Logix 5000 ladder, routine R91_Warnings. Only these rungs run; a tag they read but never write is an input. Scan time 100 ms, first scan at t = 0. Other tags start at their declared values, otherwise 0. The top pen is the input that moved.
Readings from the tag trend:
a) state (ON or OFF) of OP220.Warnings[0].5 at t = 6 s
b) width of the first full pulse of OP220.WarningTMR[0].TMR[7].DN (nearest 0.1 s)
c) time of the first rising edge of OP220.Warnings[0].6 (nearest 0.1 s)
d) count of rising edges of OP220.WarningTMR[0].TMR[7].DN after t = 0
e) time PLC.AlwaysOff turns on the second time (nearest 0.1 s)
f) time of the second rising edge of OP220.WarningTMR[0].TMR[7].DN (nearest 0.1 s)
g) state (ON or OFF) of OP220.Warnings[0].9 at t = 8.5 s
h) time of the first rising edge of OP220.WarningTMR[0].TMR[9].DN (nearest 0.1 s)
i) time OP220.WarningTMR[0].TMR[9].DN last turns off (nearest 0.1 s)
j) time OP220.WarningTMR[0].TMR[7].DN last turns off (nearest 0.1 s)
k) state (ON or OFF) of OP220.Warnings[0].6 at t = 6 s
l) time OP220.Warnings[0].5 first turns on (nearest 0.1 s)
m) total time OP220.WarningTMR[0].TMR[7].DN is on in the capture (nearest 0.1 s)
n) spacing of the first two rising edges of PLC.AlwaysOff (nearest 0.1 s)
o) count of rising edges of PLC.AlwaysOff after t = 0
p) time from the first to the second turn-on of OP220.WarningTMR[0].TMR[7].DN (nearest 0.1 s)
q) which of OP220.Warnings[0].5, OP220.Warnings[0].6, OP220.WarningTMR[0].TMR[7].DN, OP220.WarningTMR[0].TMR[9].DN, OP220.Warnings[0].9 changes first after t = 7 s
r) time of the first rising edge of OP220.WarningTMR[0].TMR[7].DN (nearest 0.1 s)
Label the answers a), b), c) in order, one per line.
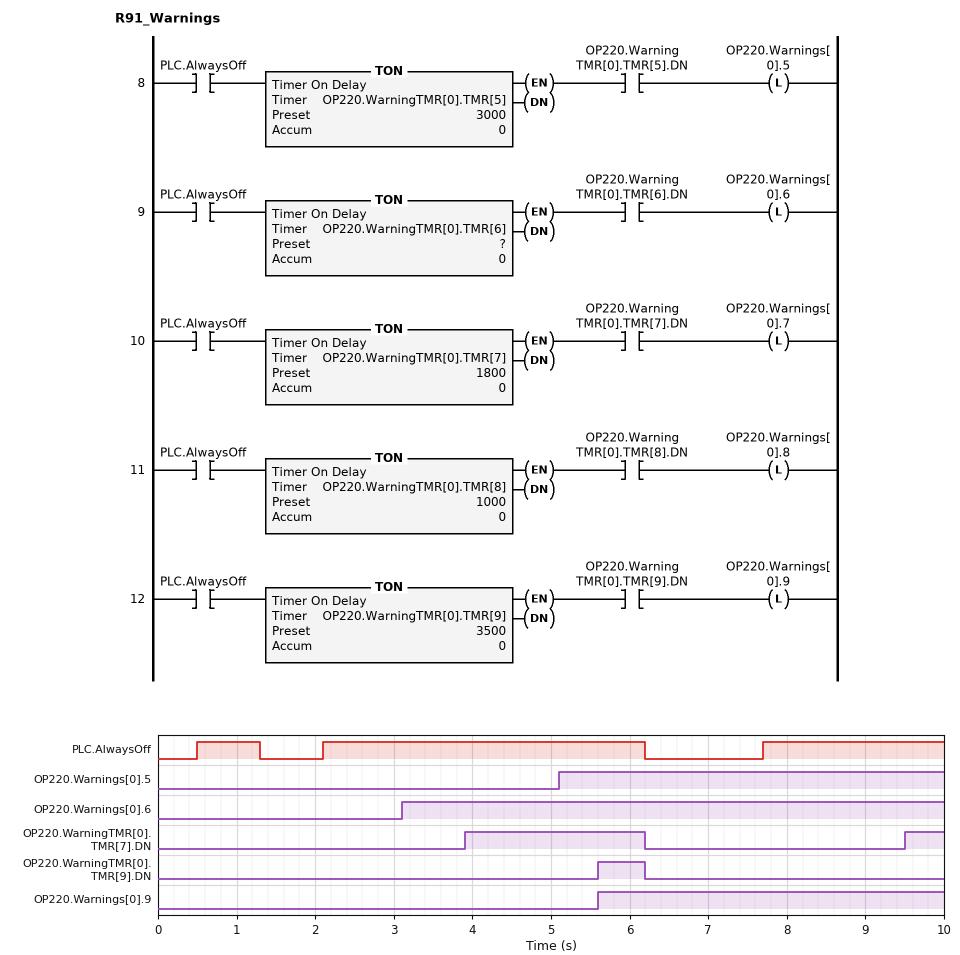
a) ON
b) 2.3 s
c) 3.1 s
d) 2
e) 2.1 s
f) 9.5 s
g) ON
h) 5.6 s
i) 6.2 s
j) 6.2 s
k) ON
l) 5.1 s
m) 2.8 s
n) 1.6 s
o) 3
p) 5.6 s
q) OP220.WarningTMR[0].TMR[7].DN
r) 3.9 s
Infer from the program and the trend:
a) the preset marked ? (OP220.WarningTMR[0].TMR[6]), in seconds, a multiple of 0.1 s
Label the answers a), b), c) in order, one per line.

a) 1.0 s
